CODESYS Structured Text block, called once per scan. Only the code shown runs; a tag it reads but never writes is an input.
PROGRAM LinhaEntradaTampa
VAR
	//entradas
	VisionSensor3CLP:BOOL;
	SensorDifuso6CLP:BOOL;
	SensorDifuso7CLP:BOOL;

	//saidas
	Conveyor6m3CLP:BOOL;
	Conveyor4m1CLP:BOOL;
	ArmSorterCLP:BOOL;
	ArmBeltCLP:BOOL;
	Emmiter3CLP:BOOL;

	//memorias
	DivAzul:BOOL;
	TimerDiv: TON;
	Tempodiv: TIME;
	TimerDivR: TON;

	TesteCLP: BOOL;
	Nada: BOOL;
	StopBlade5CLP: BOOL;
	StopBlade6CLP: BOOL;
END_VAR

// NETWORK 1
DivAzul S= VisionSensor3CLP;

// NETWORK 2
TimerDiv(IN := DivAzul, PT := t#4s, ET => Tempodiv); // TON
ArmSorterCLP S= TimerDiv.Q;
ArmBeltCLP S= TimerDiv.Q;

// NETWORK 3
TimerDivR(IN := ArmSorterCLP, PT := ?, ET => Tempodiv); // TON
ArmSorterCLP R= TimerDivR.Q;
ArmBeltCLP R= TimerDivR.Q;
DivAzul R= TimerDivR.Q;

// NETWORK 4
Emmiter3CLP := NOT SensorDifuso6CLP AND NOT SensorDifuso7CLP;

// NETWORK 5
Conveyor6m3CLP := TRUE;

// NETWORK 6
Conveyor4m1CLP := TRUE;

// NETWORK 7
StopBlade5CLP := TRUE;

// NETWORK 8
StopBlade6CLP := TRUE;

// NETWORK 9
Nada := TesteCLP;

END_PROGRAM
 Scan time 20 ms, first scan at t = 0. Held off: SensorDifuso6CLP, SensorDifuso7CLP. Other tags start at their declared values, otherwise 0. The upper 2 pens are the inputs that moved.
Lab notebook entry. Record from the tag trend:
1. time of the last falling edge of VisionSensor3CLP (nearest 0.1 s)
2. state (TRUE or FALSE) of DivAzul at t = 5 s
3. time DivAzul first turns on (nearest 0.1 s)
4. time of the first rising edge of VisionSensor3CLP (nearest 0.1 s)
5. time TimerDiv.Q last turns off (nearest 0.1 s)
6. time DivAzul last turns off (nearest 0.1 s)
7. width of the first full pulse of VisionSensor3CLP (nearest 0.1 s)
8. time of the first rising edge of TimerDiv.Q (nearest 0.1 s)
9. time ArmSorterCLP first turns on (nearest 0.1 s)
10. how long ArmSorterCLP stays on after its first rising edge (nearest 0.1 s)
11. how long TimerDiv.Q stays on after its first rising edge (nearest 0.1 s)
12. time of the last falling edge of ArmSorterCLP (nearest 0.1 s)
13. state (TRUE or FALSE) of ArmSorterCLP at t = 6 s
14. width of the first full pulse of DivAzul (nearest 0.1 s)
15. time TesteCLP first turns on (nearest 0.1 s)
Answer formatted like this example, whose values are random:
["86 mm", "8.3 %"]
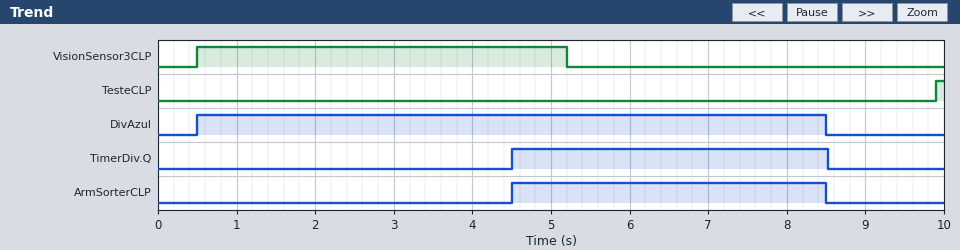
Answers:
["5.2 s", "TRUE", "0.5 s", "0.5 s", "8.5 s", "8.5 s", "4.7 s", "4.5 s", "4.5 s", "4.0 s", "4.0 s", "8.5 s", "TRUE", "8.0 s", "9.9 s"]
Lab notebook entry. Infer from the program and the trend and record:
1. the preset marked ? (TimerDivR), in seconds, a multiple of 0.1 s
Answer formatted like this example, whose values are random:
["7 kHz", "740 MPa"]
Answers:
["4.0 s"]
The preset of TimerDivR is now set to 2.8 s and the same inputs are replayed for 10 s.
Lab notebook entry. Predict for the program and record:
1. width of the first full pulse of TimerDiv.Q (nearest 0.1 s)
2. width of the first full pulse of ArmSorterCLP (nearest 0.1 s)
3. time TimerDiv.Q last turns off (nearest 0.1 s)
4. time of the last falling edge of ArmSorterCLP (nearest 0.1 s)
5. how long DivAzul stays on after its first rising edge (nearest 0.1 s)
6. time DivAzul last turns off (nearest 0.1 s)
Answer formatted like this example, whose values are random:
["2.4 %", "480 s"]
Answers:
["2.8 s", "2.8 s", "7.3 s", "7.3 s", "6.8 s", "7.3 s"]
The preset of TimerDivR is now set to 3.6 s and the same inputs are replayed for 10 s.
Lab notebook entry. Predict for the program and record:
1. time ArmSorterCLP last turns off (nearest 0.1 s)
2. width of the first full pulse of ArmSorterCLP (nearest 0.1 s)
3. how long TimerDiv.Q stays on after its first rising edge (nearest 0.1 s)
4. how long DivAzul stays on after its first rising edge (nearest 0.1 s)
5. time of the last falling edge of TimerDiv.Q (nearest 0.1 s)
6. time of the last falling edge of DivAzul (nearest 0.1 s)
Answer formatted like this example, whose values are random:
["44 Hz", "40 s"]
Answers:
["8.1 s", "3.6 s", "3.6 s", "7.6 s", "8.1 s", "8.1 s"]
